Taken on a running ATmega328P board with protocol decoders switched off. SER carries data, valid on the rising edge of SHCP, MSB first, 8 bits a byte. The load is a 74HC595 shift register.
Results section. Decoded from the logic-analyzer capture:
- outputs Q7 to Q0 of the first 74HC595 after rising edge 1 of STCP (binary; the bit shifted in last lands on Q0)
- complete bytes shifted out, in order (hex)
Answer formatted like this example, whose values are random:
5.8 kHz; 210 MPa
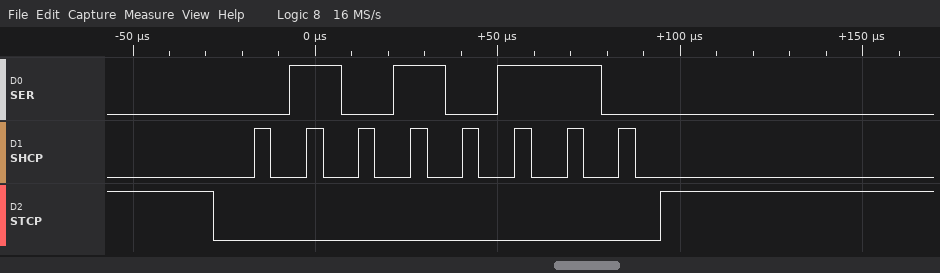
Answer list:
01010110; 56
